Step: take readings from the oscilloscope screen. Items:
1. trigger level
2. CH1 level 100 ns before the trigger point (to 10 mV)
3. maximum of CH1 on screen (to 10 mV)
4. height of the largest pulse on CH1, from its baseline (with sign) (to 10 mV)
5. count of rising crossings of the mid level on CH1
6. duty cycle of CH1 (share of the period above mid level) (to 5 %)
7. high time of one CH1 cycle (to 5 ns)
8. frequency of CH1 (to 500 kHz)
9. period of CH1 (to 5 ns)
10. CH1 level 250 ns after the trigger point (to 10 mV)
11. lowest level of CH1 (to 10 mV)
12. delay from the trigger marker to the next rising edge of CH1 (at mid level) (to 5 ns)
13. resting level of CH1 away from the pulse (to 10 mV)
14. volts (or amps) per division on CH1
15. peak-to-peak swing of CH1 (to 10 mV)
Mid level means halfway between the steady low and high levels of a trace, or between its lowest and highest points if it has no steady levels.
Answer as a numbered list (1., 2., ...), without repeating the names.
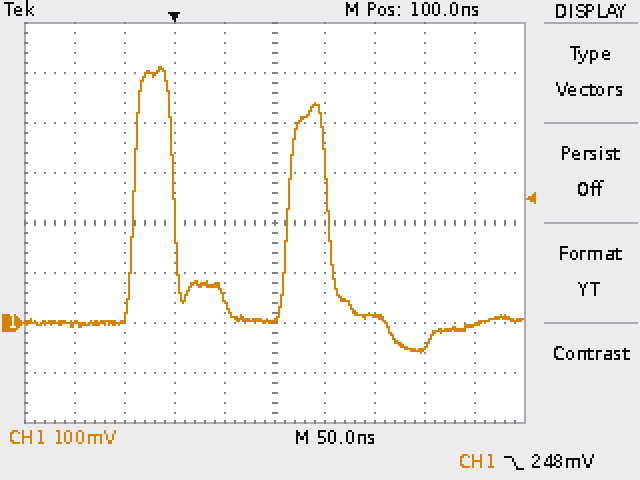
1. 248 mV
2. 0 mV
3. 510 mV
4. +510 mV
5. 2
6. 25 %
7. 40 ns
8. 6.5 MHz
9. 155 ns
10. -50 mV
11. -60 mV
12. 115 ns
13. 0 mV
14. 100 mV
15. 570 mV
